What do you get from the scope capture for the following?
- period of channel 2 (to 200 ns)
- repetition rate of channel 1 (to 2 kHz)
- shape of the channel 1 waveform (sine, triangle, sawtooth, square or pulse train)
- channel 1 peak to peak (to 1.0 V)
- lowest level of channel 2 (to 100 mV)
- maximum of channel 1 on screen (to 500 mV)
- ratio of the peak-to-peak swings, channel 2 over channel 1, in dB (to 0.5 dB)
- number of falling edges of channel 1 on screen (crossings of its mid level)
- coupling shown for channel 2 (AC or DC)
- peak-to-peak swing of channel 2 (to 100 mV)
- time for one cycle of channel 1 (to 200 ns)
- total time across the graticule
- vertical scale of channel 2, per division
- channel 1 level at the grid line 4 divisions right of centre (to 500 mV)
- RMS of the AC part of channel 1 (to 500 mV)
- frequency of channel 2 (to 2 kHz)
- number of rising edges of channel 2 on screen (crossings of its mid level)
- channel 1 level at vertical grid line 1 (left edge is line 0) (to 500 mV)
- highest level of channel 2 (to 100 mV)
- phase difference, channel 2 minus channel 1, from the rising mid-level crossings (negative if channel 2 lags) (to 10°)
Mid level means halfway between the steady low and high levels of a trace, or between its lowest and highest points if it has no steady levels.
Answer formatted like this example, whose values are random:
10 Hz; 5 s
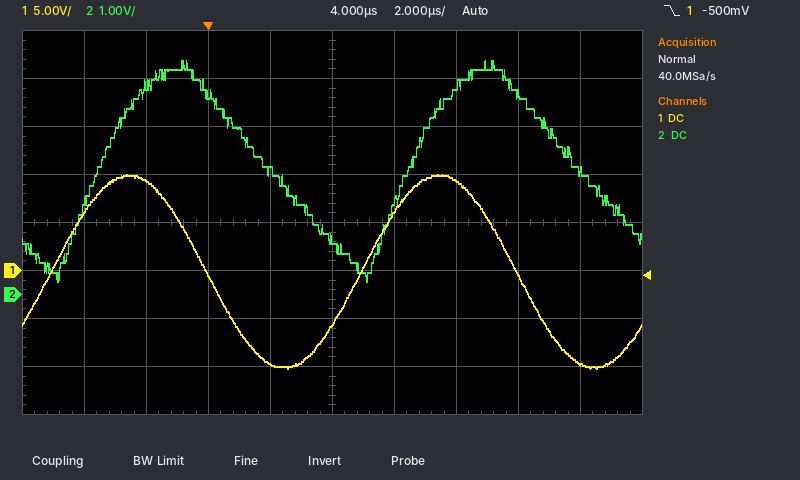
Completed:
10.0 µs; 100 kHz; sine; 20.0 V; 300 mV; 10.0 V; -13.0 dB; 2; DC; 4.6 V; 10.0 µs; 20 µs; 1 V; -9.5 V; 7.0 V; 100 kHz; 2; 6.0 V; 4.9 V; -50°
